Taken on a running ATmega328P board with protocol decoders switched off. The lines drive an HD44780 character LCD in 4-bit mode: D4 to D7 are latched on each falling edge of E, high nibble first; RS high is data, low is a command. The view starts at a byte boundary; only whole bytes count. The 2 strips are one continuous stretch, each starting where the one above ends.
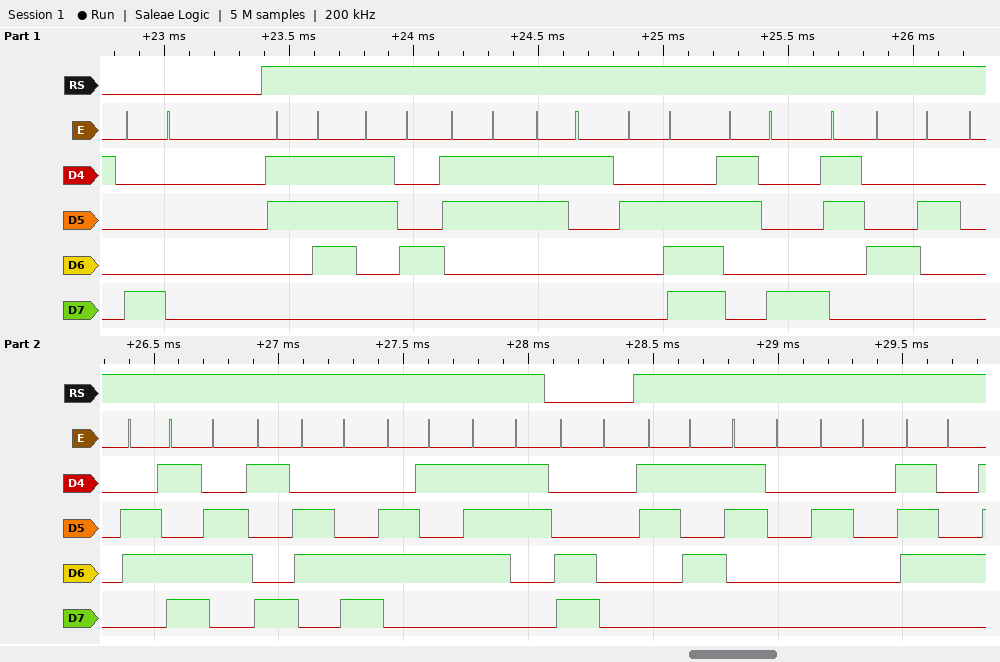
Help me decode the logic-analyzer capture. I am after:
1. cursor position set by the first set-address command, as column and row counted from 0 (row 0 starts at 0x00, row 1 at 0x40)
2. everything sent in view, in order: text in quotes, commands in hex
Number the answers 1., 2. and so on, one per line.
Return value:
1. column 0, row 0
2. 0x80 "7431.84 miles" 0xC0 "50 t"
